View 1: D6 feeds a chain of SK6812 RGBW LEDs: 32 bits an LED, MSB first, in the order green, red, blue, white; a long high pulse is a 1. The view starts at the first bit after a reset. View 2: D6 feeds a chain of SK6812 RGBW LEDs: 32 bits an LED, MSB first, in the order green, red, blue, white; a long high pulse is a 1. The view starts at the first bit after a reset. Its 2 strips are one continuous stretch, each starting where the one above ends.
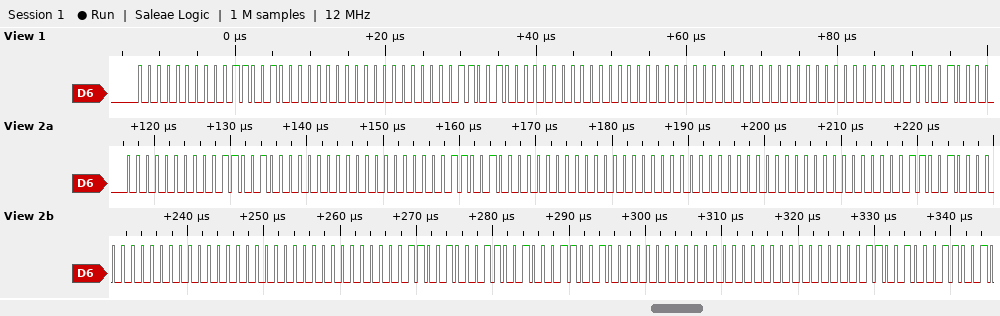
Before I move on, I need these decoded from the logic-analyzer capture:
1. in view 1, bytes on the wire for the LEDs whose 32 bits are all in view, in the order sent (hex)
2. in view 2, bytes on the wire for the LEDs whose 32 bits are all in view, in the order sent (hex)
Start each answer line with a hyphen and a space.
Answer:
- 00 32 00 00 32 00 00 00
- 00 32 00 00 32 00 00 00 00 00 32 00 00 00 00 32 32 32 00 00
